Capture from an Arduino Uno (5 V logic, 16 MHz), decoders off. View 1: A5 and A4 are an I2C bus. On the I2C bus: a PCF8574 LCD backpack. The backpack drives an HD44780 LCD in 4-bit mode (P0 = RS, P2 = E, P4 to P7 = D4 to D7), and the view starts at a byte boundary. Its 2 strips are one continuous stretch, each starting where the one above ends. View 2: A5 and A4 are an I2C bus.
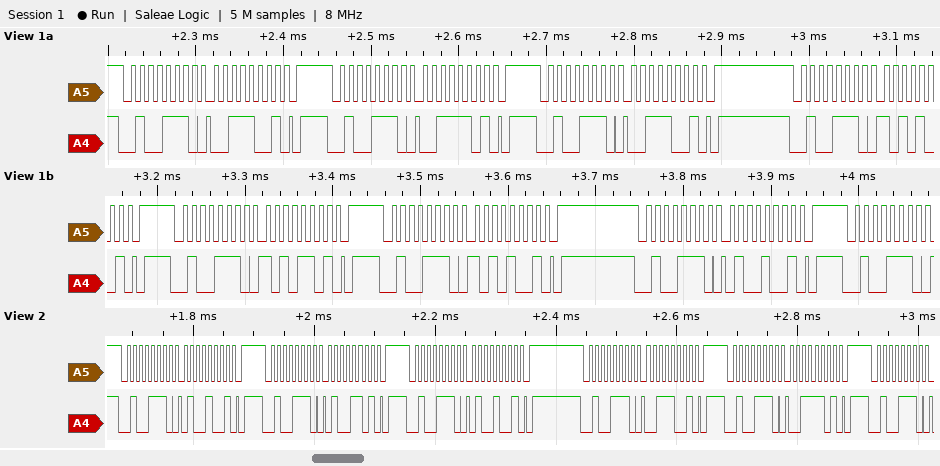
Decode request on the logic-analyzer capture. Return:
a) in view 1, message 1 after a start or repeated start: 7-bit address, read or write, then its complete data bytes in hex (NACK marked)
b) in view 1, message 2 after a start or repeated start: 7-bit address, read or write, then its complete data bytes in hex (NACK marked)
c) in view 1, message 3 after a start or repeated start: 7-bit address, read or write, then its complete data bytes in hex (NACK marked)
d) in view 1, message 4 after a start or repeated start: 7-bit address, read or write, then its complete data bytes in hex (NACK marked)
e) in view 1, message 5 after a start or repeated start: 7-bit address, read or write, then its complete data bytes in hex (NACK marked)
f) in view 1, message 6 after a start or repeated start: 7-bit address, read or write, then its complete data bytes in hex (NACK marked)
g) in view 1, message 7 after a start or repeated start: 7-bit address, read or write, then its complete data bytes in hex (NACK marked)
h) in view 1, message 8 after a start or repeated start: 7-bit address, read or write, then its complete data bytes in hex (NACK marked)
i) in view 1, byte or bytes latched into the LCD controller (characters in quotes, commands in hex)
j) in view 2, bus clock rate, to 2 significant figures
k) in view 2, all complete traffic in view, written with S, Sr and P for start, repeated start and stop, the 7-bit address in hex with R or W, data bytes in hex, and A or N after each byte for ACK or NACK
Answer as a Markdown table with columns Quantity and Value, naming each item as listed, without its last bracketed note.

| Quantity | Value |
|---|---|
| in view 1, message 1 after a start or repeated start: 7-bit address, read or write, then its complete data bytes in hex | 0x27 write: 39 |
| in view 1, message 2 after a start or repeated start: 7-bit address, read or write, then its complete data bytes in hex | 0x27 write: 3D |
| in view 1, message 3 after a start or repeated start: 7-bit address, read or write, then its complete data bytes in hex | 0x27 write: 39 |
| in view 1, message 4 after a start or repeated start: 7-bit address, read or write, then its complete data bytes in hex | 0x27 write: A9 |
| in view 1, message 5 after a start or repeated start: 7-bit address, read or write, then its complete data bytes in hex | 0x27 write: AD |
| in view 1, message 6 after a start or repeated start: 7-bit address, read or write, then its complete data bytes in hex | 0x27 write: A9 |
| in view 1, message 7 after a start or repeated start: 7-bit address, read or write, then its complete data bytes in hex | 0x27 write: 49 |
| in view 1, message 8 after a start or repeated start: 7-bit address, read or write, then its complete data bytes in hex | 0x27 write |
| in view 1, byte or bytes latched into the LCD controller | ':' |
| in view 2, bus clock rate, to 2 significant figures | 100 kHz |
| in view 2, all complete traffic in view, written with S, Sr and P for start, repeated start and stop, the 7-bit address in hex with R or W, data bytes in hex, and A or N after each byte for ACK or NACK | S 27W A 49 A P S 27W A 4D A P S 27W A 49 A P S 27W A 39 A P S 27W A 3D A P S 27W A |
